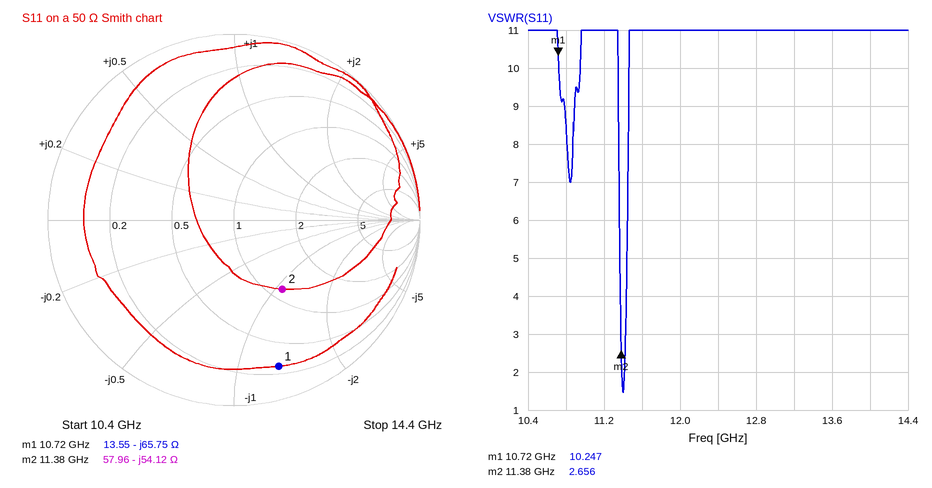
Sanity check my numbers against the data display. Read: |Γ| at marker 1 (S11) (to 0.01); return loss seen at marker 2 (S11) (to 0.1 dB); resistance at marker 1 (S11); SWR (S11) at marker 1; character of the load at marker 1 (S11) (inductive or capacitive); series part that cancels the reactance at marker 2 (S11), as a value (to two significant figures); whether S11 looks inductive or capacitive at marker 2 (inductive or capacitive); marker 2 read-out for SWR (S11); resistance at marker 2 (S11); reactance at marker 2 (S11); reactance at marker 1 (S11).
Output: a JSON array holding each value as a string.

["0.82", "6.9 dB", "13.55 Ω", "10.247", "capacitive", "760 pH", "capacitive", "2.656", "57.96 Ω", "-54.12 Ω", "-65.75 Ω"]
